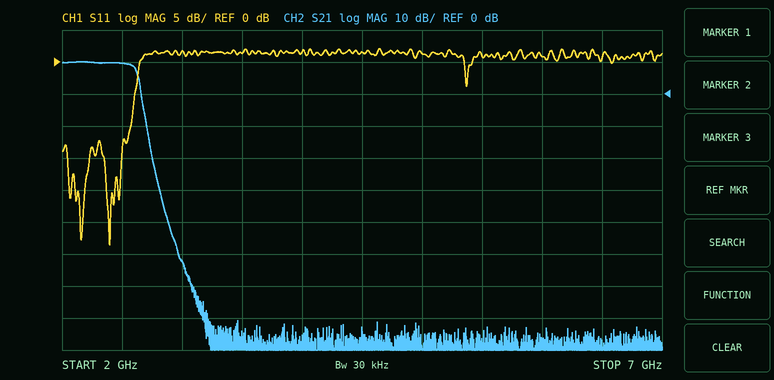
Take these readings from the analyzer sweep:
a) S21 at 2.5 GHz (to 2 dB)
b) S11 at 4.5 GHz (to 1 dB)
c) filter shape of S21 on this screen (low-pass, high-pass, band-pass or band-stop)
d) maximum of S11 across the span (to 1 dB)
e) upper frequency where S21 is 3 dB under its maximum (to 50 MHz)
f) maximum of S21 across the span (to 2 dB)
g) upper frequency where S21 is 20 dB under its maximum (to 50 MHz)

10 dB
2 dB
low-pass
2 dB
2.60 GHz
10 dB
2.70 GHz
